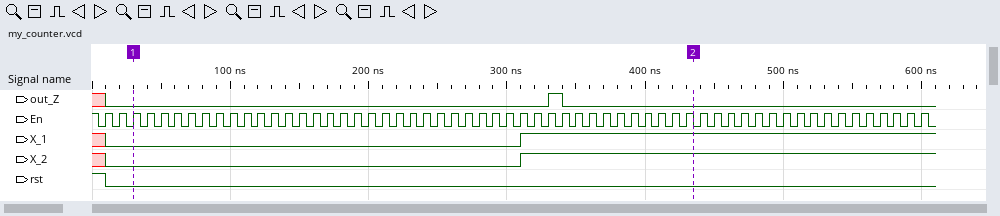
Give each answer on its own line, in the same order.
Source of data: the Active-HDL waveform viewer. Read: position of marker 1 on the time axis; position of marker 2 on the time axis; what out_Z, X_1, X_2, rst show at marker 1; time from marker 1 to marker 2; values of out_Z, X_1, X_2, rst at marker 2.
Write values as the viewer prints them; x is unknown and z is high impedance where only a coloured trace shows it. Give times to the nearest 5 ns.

30 ns
435 ns
out_Z=0, X_1=0, X_2=0, rst=0
405 ns
out_Z=0, X_1=1, X_2=1, rst=0
